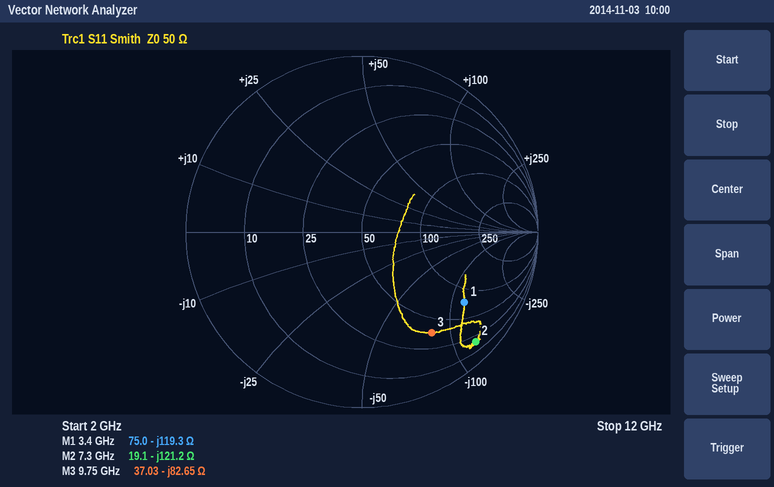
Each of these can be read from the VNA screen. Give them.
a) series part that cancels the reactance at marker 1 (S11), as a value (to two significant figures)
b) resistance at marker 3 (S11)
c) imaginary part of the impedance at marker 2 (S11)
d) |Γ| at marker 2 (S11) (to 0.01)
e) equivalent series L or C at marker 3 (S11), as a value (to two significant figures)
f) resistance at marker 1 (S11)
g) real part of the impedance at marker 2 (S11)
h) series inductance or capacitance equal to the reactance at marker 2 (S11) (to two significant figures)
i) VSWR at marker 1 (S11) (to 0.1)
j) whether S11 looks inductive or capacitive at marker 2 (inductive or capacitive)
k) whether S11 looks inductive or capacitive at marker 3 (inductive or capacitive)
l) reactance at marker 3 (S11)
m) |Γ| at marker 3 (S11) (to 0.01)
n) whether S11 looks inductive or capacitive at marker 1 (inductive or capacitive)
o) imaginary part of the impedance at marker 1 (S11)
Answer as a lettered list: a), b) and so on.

a) 5.6 nH
b) 37.03 Ω
c) -121.2 Ω
d) 0.90
e) 200 fF
f) 75.0 Ω
g) 19.1 Ω
h) 180 fF
i) 5.8
j) capacitive
k) capacitive
l) -82.65 Ω
m) 0.70
n) capacitive
o) -119.3 Ω
